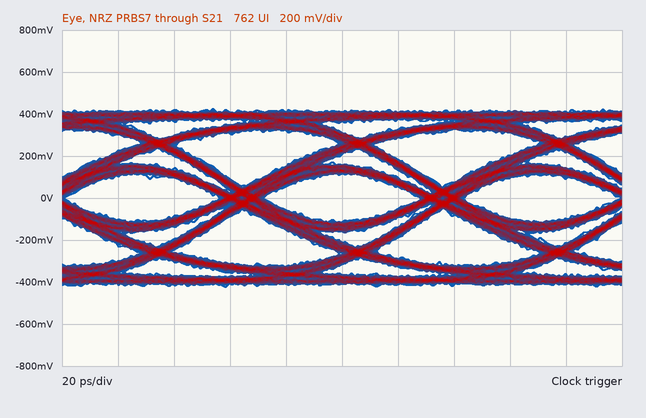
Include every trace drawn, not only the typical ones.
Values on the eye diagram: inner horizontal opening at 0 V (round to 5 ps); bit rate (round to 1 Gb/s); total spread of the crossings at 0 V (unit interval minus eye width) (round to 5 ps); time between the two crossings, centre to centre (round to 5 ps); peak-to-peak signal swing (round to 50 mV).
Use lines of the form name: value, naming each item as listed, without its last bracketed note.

inner horizontal opening at 0 V: 55 ps
bit rate: 14 Gb/s
total spread of the crossings at 0 V (unit interval minus eye width): 15 ps
time between the two crossings, centre to centre: 70 ps
peak-to-peak signal swing: 850 mV
